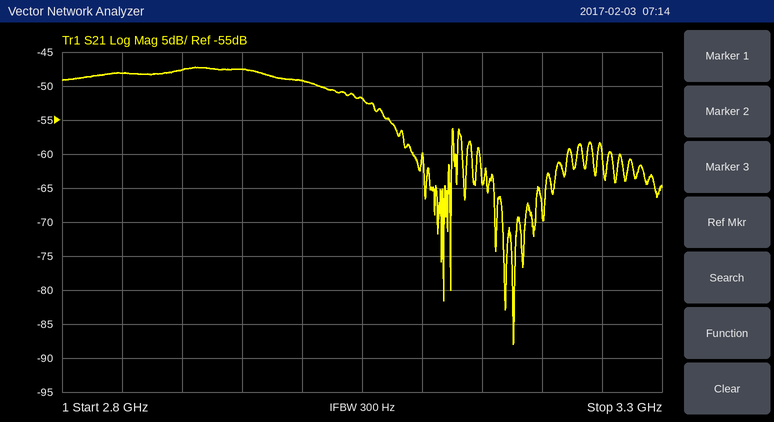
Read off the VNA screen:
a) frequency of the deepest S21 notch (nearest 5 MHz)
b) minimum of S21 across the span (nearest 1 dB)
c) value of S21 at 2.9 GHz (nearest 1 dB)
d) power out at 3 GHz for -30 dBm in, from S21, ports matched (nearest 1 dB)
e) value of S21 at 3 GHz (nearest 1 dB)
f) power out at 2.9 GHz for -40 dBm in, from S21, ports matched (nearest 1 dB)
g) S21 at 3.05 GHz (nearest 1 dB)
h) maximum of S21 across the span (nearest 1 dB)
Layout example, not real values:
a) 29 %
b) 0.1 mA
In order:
a) 3.175 GHz
b) -88 dB
c) -48 dB
d) -79 dBm
e) -49 dB
f) -88 dBm
g) -52 dB
h) -47 dB
